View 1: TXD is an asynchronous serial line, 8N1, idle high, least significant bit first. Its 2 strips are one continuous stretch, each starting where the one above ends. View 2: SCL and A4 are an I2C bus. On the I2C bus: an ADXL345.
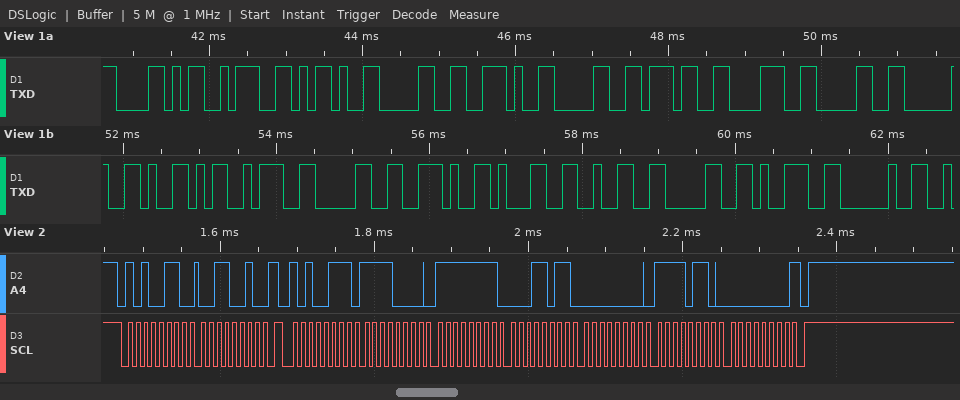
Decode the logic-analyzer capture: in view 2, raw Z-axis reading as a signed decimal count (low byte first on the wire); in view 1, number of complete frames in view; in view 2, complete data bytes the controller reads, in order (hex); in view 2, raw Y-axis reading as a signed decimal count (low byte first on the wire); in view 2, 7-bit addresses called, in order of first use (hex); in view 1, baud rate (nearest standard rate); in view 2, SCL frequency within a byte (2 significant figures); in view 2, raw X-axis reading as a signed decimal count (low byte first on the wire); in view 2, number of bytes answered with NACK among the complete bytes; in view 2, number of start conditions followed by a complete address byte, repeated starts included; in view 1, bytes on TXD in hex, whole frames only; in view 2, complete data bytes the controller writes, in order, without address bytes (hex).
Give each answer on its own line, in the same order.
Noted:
246
19
F0 FF 1B 00 F6 00
27
0x53
9600 baud
100 kHz
-16
1
2
58 3A 2D 30 2E 30 37 38 30 20 59 3A 30 2E 31 32 30 39 20
32
